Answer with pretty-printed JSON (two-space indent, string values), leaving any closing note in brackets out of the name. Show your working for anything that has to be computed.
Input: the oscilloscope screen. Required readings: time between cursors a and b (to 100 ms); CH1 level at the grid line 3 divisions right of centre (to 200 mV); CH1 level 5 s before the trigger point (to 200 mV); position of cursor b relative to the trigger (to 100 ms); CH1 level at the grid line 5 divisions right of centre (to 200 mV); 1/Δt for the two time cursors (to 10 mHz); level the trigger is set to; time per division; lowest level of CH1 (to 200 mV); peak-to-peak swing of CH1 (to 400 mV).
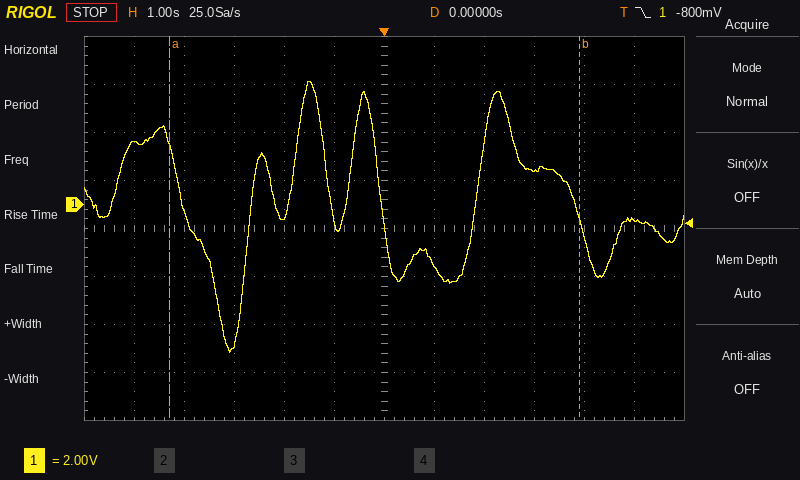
{
  "time between cursors a and b": "8.2 s",
  "CH1 level at the grid line 3 divisions right of centre": "1.4 V",
  "CH1 level 5 s before the trigger point": "2.6 V",
  "position of cursor b relative to the trigger": "+3.9 s",
  "CH1 level at the grid line 5 divisions right of centre": "-600 mV",
  "1/Δt for the two time cursors": "1 / 8.2 s ≈ 120 mHz",
  "level the trigger is set to": "-800 mV",
  "time per division": "1 s",
  "lowest level of CH1": "-6.2 V",
  "peak-to-peak swing of CH1": "11.2 V"
}
